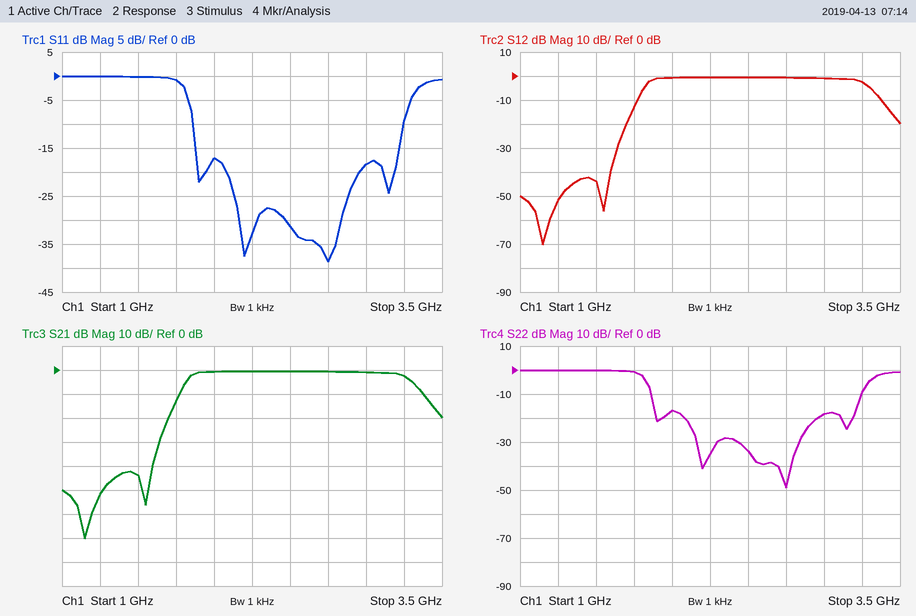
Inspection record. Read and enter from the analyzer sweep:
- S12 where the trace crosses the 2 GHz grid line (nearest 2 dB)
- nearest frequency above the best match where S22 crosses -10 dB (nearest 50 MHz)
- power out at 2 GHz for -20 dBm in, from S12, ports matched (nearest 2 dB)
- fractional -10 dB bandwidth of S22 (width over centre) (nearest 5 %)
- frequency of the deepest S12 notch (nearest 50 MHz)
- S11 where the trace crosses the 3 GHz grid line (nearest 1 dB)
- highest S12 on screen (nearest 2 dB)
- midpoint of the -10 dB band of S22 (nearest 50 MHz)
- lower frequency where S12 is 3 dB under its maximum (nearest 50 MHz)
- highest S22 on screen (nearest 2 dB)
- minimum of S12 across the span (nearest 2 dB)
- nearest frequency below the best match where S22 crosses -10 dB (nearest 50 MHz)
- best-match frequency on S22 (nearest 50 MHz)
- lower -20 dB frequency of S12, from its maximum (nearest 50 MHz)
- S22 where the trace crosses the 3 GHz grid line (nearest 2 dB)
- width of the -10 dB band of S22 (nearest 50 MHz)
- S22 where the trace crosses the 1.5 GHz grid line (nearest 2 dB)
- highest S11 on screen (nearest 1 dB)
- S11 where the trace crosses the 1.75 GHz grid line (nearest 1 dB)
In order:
0 dB
3.25 GHz
-20 dBm
55 %
1.15 GHz
-18 dB
0 dB
2.55 GHz
1.85 GHz
0 dB
-70 dB
1.85 GHz
2.75 GHz
1.70 GHz
-18 dB
1.40 GHz
0 dB
0 dB
-1 dB
